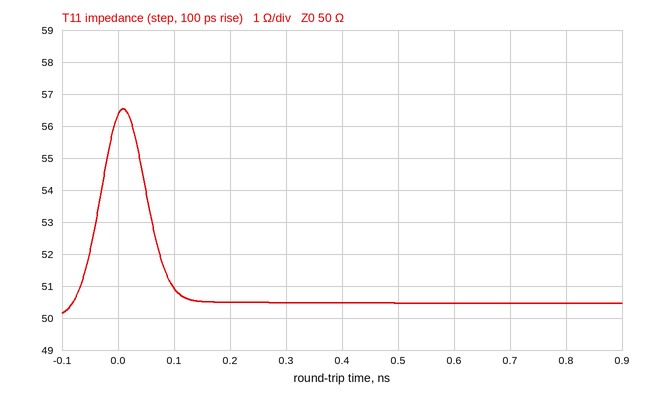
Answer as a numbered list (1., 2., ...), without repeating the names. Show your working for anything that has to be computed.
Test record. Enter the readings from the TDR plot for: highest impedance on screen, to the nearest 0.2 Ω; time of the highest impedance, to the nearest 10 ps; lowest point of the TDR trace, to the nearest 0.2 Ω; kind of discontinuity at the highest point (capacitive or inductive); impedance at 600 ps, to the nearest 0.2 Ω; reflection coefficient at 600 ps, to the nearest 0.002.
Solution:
1. 56.6 Ω
2. 10 ps
3. 50.2 Ω
4. inductive
5. 50.4 Ω
6. (50.4 − 50)/(50.4 + 50) ≈ +0.004
